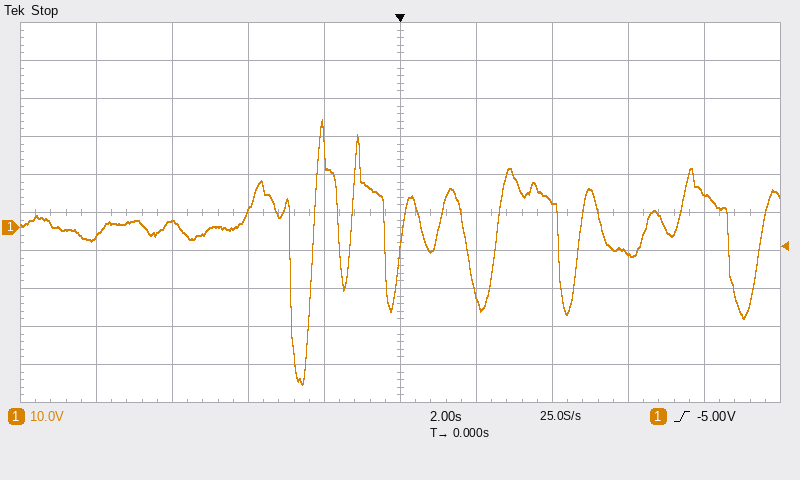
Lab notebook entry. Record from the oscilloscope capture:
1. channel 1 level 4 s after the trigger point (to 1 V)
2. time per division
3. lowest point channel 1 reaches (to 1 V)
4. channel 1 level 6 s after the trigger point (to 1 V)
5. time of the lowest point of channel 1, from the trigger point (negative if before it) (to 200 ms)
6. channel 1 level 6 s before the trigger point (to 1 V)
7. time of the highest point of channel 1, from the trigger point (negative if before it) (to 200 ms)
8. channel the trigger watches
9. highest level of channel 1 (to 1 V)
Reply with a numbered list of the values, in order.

1. 7 V
2. 2 s
3. -41 V
4. -7 V
5. -2.6 s
6. 2 V
7. -2.0 s
8. channel 1
9. 28 V
